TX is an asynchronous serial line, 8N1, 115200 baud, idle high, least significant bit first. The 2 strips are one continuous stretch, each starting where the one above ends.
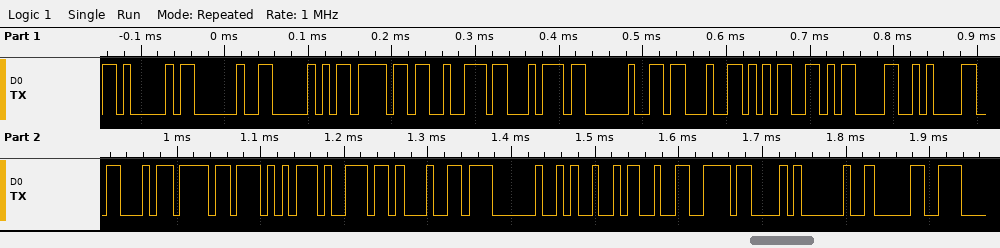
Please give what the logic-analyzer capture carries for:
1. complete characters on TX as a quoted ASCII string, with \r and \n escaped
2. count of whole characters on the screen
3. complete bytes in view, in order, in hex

"A Port #5\r\nFound I2C 0"
22
41 20 50 6F 72 74 20 23 35 0D 0A 46 6F 75 6E 64 20 49 32 43 20 30
